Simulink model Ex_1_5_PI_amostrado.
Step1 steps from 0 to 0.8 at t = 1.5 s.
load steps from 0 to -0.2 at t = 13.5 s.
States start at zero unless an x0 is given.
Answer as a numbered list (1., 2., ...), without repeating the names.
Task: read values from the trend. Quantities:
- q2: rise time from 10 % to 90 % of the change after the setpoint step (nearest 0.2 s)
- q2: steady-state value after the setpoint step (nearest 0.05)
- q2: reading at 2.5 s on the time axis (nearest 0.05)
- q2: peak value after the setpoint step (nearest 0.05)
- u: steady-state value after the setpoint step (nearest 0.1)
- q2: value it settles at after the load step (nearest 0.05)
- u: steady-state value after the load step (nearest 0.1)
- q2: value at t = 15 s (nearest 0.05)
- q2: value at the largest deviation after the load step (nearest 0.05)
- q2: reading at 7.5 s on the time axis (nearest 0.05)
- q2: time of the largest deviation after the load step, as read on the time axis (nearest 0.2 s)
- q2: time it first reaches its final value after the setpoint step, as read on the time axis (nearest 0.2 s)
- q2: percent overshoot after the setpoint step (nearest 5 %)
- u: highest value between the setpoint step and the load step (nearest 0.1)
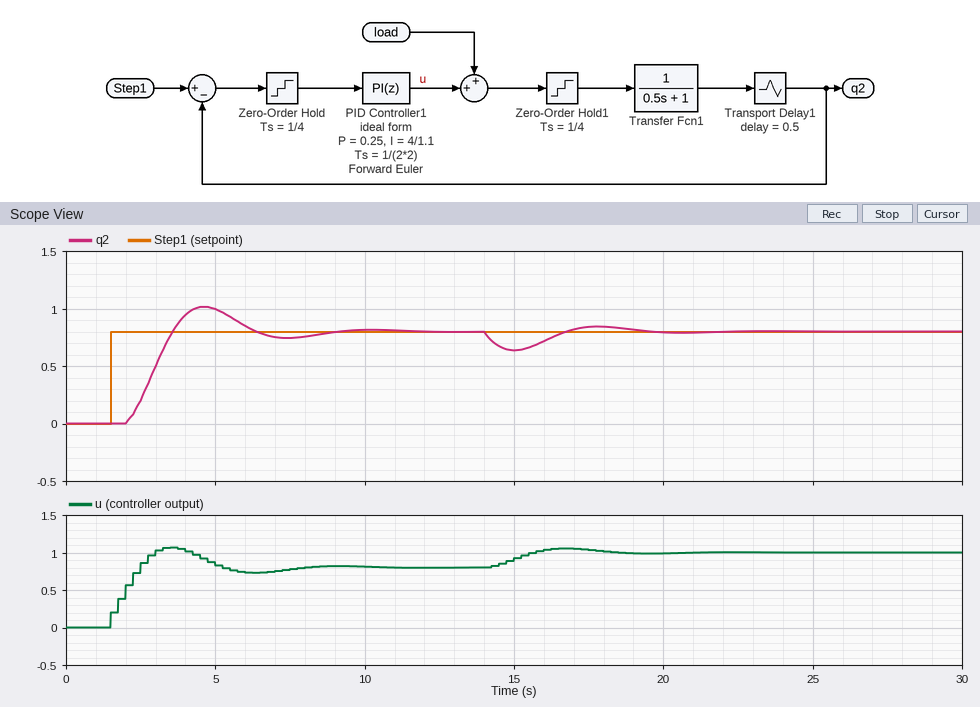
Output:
1. 1.2 s
2. 0.80
3. 0.20
4. 1.00
5. 0.8
6. 0.80
7. 1.0
8. 0.65
9. 0.65
10. 0.75
11. 15.0 s
12. 3.6 s
13. 25 %
14. 1.1
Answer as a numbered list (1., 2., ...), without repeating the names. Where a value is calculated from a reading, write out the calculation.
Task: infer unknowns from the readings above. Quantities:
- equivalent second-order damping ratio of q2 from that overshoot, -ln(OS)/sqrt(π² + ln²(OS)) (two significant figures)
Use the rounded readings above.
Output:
1. ln(0.25) = -1.386; 1.386 / sqrt(9.870 + 1.922) = 0.40
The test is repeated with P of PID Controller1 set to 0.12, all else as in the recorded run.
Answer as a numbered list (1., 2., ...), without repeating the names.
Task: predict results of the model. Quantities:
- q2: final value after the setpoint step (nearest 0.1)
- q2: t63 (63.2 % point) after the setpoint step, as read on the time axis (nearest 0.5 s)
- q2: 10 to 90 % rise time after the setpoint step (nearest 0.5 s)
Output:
1. 0.8
2. 4.0 s
3. 3.0 s
